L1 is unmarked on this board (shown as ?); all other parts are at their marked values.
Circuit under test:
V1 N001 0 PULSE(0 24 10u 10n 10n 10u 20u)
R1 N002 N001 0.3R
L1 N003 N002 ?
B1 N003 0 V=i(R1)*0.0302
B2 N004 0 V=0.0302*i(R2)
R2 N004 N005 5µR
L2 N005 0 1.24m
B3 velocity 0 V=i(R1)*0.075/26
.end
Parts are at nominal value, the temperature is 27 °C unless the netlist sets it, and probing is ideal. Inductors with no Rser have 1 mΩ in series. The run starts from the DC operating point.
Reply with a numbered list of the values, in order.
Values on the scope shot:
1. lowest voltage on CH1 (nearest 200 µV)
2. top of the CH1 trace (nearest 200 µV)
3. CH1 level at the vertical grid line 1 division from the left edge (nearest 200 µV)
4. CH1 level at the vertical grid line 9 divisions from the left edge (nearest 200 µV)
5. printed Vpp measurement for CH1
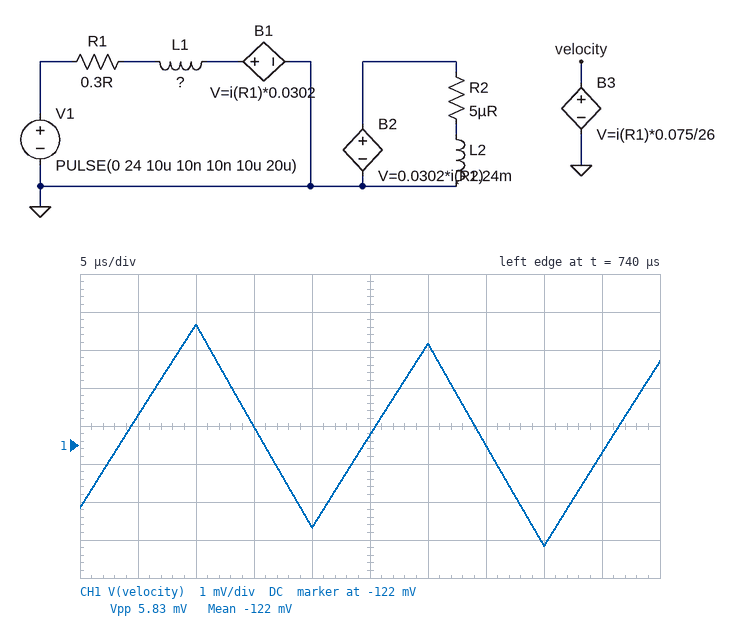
1. -124.6 mV
2. -118.8 mV
3. -121.2 mV
4. -122.2 mV
5. 5.83 mV
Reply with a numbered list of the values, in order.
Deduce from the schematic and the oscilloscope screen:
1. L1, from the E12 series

1. 68 µH
